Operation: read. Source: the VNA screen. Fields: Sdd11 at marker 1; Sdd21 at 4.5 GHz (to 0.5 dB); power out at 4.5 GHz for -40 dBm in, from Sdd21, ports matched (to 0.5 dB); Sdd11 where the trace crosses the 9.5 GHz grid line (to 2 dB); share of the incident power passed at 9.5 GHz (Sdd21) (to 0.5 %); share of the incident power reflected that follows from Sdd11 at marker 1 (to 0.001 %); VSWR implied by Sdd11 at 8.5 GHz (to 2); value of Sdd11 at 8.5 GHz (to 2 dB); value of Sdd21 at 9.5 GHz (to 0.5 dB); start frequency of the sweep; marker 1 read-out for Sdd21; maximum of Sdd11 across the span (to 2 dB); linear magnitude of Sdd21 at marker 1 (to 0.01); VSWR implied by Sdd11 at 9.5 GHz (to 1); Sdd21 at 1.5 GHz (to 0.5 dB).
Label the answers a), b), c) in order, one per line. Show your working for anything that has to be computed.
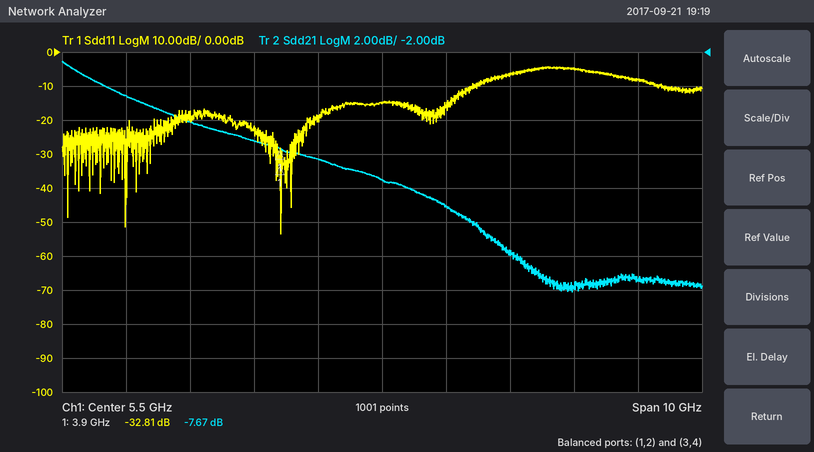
a) -32.81 dB
b) -8.5 dB
c) -40 dBm + (-8.5 dB) = -48.5 dBm
d) -8 dB
e) 10^(-15.5/10) ≈ 2.82 %, so 3.0 % to the nearest 0.5 %
f) 10^(-32.81/10) ≈ 0.052 %
g) |Γ| = 10^(-4/20) = 0.6310; VSWR = (1 + 0.6310)/(1 − 0.6310) ≈ 4
h) -4 dB
i) -15.5 dB
j) 500 MHz
k) -7.67 dB
l) -4 dB
m) 10^(-7.67/20) ≈ 0.41
n) |Γ| = 10^(-8/20) = 0.3981; VSWR = (1 + 0.3981)/(1 − 0.3981) ≈ 2
o) -4.5 dB
